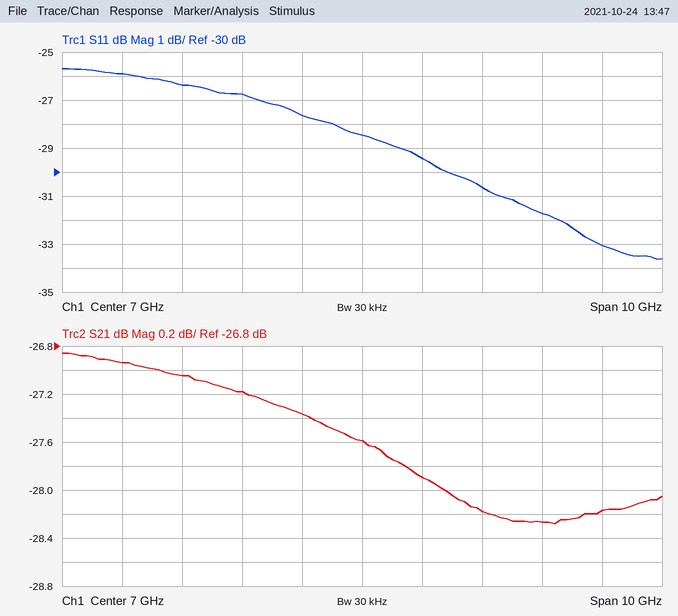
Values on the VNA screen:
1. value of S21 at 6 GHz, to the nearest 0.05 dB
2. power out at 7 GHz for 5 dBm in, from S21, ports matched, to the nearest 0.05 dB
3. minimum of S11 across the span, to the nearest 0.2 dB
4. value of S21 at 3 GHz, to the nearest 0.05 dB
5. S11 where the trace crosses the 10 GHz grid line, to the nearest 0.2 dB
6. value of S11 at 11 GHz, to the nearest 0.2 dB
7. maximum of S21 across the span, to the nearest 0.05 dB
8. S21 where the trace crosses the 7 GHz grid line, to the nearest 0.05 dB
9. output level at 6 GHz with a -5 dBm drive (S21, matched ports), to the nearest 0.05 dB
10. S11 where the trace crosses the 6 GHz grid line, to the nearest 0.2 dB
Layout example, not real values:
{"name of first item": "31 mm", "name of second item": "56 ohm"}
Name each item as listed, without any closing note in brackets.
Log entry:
{"value of S21 at 6 GHz, to the nearest 0.05 dB": "-27.35 dB", "power out at 7 GHz for 5 dBm in, from S21, ports matched, to the nearest 0.05 dB": "-22.60 dBm", "minimum of S11 across the span, to the nearest 0.2 dB": "-33.6 dB", "value of S21 at 3 GHz, to the nearest 0.05 dB": "-26.95 dB", "S11 where the trace crosses the 10 GHz grid line, to the nearest 0.2 dB": "-31.8 dB", "value of S11 at 11 GHz, to the nearest 0.2 dB": "-33.0 dB", "maximum of S21 across the span, to the nearest 0.05 dB": "-26.85 dB", "S21 where the trace crosses the 7 GHz grid line, to the nearest 0.05 dB": "-27.60 dB", "output level at 6 GHz with a -5 dBm drive (S21, matched ports), to the nearest 0.05 dB": "-32.35 dBm", "S11 where the trace crosses the 6 GHz grid line, to the nearest 0.2 dB": "-27.6 dB"}
